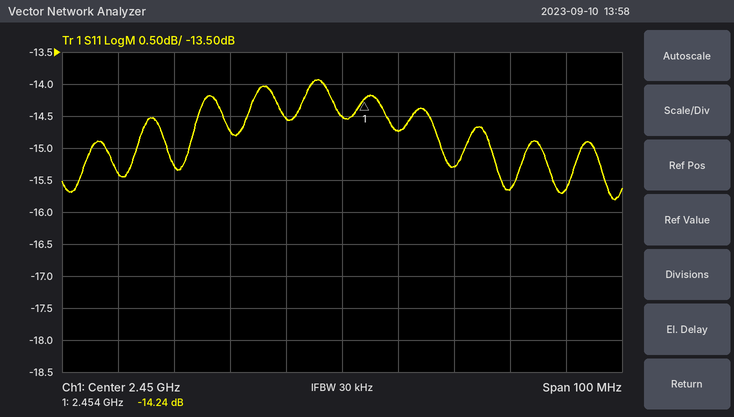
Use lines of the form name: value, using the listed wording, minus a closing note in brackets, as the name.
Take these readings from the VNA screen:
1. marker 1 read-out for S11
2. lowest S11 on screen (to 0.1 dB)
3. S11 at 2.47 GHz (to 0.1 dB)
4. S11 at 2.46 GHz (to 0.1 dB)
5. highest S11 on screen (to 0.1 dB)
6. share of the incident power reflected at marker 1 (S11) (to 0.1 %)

marker 1 read-out for S11: -14.24 dB
lowest S11 on screen: -15.8 dB
S11 at 2.47 GHz: -15.3 dB
S11 at 2.46 GHz: -14.7 dB
highest S11 on screen: -13.9 dB
share of the incident power reflected at marker 1 (S11): 3.8 %
